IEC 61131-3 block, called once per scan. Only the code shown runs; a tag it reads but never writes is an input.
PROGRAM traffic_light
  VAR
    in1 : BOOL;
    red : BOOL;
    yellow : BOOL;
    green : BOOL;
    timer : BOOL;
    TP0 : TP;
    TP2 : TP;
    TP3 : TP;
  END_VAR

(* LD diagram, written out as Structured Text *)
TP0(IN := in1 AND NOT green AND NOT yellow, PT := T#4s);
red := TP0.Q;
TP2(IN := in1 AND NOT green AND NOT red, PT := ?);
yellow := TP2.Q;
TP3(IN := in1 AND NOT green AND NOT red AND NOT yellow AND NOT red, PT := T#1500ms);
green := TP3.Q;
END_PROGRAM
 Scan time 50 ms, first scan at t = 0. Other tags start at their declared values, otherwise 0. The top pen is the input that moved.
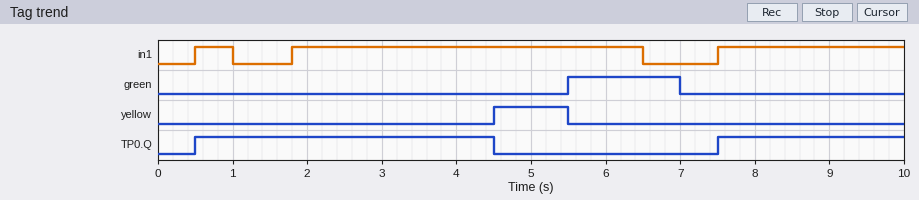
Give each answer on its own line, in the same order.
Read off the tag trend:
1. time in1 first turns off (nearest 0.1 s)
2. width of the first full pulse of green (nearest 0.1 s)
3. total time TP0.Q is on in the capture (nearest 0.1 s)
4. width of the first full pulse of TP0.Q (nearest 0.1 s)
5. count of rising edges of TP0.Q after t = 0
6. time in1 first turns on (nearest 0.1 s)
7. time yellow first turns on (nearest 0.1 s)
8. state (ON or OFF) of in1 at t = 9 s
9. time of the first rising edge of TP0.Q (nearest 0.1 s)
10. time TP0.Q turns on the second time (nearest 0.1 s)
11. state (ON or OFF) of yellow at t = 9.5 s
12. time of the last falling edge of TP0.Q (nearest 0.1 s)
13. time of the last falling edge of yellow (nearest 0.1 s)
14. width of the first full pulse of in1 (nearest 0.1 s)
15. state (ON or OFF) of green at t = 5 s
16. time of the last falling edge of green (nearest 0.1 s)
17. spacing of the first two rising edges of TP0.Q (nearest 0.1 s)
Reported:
1.0 s
1.5 s
6.5 s
4.0 s
2
0.5 s
4.5 s
ON
0.5 s
7.5 s
OFF
4.5 s
5.5 s
0.5 s
OFF
7.0 s
7.0 s
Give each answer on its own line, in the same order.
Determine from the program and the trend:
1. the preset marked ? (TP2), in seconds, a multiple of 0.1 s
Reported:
1.0 s
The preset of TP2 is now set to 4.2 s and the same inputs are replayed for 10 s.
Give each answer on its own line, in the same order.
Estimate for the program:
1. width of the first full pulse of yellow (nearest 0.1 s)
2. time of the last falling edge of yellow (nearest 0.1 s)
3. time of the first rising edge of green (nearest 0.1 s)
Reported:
4.2 s
8.7 s
8.7 s
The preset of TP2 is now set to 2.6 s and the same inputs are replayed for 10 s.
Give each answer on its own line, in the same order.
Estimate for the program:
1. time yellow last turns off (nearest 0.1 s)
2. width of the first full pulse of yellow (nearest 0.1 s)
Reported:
7.1 s
2.6 s
